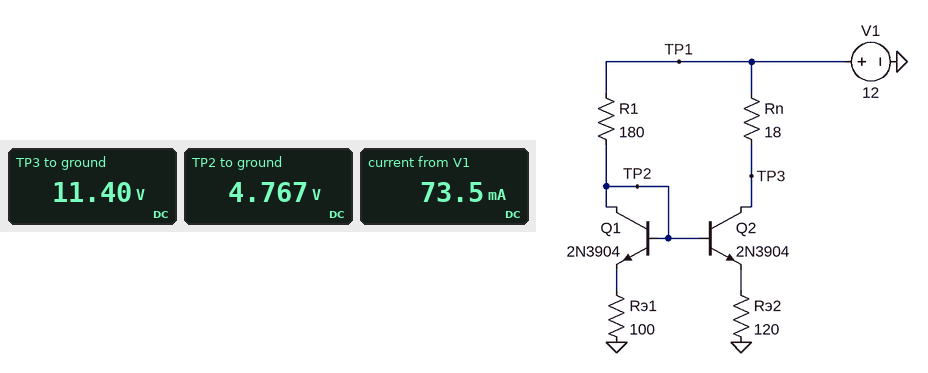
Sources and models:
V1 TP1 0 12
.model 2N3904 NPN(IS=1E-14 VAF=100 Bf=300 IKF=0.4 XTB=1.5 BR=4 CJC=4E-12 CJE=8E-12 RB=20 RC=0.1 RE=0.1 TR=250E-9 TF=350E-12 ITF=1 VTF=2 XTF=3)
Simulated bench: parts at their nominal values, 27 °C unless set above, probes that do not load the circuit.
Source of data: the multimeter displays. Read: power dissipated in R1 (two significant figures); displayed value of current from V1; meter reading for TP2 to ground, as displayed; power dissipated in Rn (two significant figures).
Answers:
290 mW
73.5 mA
4.767 V
20 mW
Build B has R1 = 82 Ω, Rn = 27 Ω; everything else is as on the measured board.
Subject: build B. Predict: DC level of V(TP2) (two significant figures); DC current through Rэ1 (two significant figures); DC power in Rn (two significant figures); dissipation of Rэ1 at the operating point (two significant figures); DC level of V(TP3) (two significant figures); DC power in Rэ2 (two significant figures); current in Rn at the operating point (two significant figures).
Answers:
6.9 V
62 mA
71 mW
380 mW
11 V
320 mW
51 mA
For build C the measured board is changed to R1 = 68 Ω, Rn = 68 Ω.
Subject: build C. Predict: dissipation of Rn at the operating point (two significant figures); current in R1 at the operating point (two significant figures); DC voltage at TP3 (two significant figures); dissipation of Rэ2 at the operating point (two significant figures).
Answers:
210 mW
67 mA
8.2 V
370 mW
